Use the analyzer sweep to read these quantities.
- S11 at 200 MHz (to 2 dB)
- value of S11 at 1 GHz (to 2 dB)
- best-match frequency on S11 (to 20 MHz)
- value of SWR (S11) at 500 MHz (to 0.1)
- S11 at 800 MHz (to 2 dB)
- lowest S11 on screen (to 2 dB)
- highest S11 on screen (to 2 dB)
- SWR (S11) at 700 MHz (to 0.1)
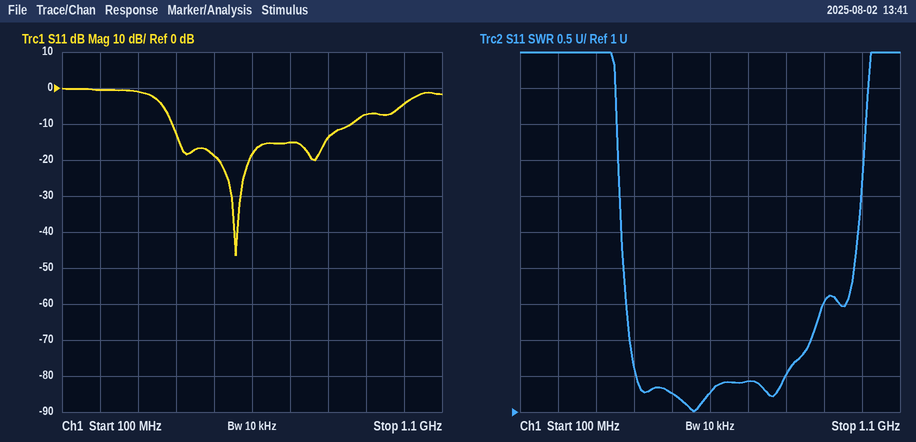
0 dB
-4 dB
560 MHz
1.3
-14 dB
-46 dB
0 dB
1.4
